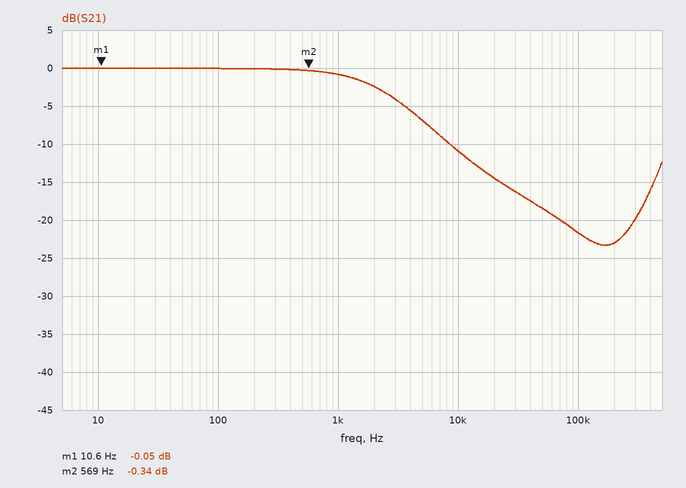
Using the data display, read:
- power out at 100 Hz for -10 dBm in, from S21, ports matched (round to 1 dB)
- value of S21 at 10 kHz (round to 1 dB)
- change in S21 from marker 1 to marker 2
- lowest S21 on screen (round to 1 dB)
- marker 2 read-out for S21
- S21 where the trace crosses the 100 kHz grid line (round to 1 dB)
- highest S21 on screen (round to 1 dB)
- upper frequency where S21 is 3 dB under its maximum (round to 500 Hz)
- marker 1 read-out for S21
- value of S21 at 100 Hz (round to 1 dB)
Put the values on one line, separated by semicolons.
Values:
-10 dBm; -11 dB; -0.29 dB; -23 dB; -0.34 dB; -22 dB; 0 dB; 2.5 kHz; -0.05 dB; 0 dB
